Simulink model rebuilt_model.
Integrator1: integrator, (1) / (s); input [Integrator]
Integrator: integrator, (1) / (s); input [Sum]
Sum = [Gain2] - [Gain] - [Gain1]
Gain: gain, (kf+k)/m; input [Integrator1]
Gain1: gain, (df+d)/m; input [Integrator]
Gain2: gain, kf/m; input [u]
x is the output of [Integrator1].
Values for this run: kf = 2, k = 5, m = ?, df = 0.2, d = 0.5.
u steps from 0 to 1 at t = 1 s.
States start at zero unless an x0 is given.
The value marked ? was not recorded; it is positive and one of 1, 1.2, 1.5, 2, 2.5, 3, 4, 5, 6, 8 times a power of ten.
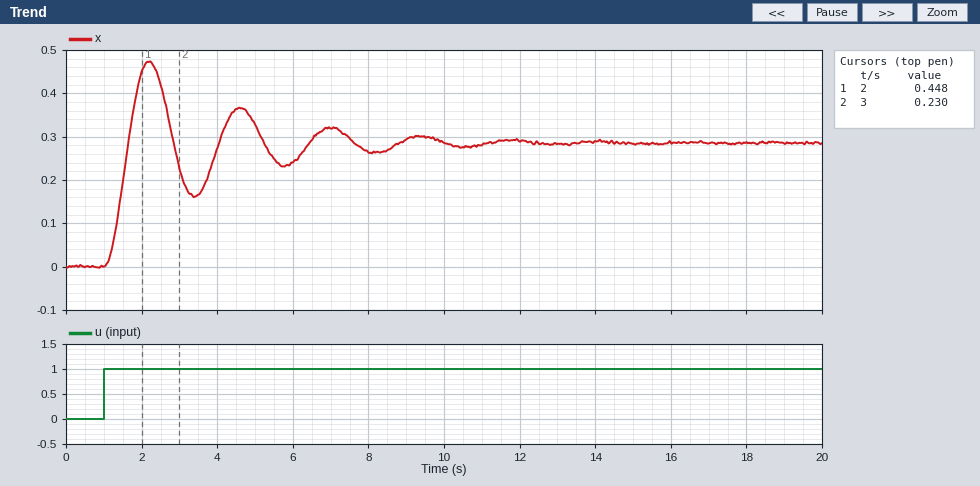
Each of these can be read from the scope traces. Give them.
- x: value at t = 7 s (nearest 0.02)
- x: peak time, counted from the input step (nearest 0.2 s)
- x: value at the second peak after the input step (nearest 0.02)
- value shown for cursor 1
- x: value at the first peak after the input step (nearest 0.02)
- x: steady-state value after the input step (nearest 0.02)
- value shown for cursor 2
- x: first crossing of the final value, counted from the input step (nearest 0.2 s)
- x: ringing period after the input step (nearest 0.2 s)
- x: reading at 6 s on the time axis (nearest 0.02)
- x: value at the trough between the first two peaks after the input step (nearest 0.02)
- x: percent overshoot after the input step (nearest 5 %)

0.32
1.2 s
0.36
0.448
0.48
0.28
0.230
0.6 s
2.4 s
0.24
0.16
65 %
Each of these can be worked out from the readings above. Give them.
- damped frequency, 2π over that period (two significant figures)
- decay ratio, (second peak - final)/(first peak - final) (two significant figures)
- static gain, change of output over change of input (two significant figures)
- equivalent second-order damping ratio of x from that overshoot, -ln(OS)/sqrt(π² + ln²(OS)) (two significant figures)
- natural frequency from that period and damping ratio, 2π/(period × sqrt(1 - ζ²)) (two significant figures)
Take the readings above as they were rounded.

2.6 rad/s
0.40
0.28
0.14
2.6 rad/s
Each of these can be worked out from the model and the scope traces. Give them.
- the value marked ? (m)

1
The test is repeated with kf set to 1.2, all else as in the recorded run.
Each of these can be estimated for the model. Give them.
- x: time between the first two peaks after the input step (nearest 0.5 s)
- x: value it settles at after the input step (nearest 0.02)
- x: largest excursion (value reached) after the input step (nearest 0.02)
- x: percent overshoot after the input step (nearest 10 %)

2.5 s
0.20
0.32
60 %
